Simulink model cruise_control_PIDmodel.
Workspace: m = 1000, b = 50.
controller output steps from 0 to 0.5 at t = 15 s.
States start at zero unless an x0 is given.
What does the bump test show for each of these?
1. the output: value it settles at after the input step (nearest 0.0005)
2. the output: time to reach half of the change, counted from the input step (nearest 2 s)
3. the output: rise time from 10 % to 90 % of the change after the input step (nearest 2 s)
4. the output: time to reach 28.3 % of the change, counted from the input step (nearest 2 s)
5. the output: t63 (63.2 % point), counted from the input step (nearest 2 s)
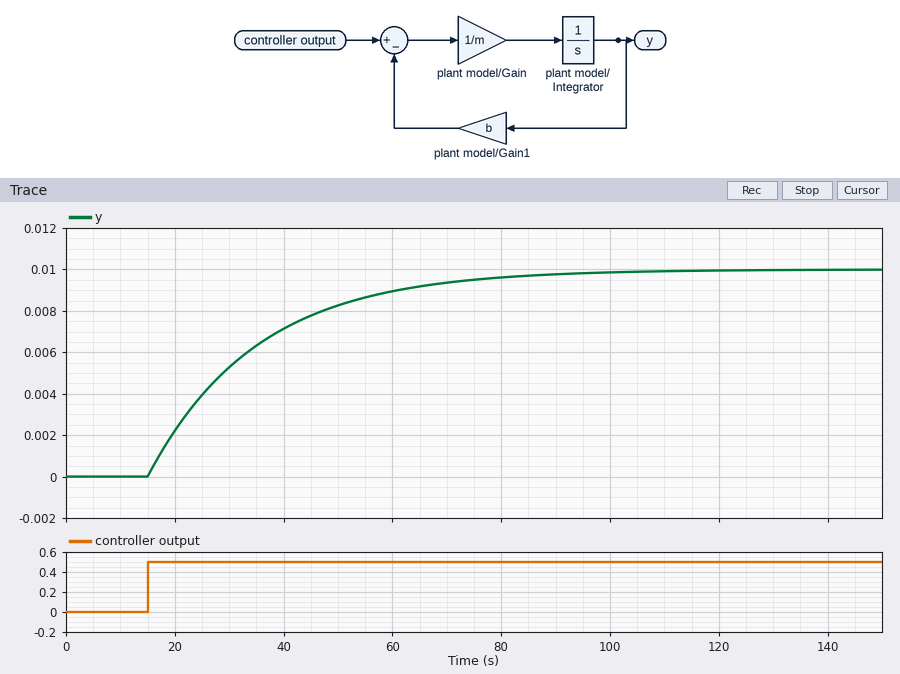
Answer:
0.0100
14 s
44 s
6 s
20 s
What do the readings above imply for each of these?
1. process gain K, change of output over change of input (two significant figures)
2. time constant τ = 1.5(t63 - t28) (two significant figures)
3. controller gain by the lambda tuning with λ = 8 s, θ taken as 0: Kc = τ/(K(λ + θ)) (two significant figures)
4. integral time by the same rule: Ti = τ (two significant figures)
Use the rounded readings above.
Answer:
0.020
21 s
130
21 s
